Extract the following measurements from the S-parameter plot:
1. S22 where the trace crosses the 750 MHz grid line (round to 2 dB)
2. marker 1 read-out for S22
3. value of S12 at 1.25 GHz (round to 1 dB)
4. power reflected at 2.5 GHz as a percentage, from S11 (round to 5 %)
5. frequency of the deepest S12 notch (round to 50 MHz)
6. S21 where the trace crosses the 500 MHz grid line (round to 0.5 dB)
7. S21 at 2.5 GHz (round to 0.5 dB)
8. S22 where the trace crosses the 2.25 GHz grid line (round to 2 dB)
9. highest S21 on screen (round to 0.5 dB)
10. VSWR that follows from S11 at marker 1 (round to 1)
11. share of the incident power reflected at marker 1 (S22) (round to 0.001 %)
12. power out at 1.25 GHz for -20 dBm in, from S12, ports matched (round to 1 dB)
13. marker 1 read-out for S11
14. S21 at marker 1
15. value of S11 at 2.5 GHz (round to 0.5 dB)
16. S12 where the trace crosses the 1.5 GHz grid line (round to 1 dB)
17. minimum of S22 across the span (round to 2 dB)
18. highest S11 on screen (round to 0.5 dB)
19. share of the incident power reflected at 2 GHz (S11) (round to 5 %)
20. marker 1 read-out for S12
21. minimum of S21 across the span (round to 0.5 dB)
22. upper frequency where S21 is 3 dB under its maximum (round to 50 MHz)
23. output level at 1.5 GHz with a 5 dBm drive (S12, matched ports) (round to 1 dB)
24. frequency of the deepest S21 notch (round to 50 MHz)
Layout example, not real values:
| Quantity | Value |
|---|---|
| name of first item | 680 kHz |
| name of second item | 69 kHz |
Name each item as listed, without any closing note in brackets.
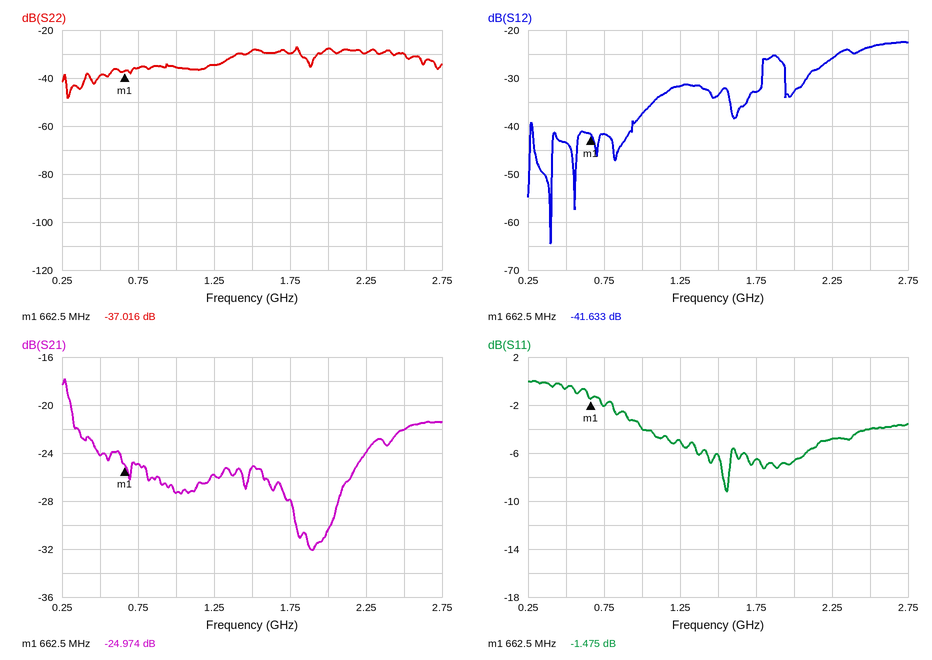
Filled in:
| Quantity | Value |
|---|---|
| S22 where the trace crosses the 750 MHz grid line | -36 dB |
| marker 1 read-out for S22 | -37.016 dB |
| value of S12 at 1.25 GHz | -32 dB |
| power reflected at 2.5 GHz as a percentage, from S11 | 40 % |
| frequency of the deepest S12 notch | 400 MHz |
| S21 where the trace crosses the 500 MHz grid line | -24.0 dB |
| S21 at 2.5 GHz | -22.0 dB |
| S22 where the trace crosses the 2.25 GHz grid line | -30 dB |
| highest S21 on screen | -18.0 dB |
| VSWR that follows from S11 at marker 1 | 12 |
| share of the incident power reflected at marker 1 (S22) | 0.020 % |
| power out at 1.25 GHz for -20 dBm in, from S12, ports matched | -52 dBm |
| marker 1 read-out for S11 | -1.475 dB |
| S21 at marker 1 | -24.974 dB |
| value of S11 at 2.5 GHz | -4.0 dB |
| S12 where the trace crosses the 1.5 GHz grid line | -34 dB |
| minimum of S22 across the span | -48 dB |
| highest S11 on screen | 0.0 dB |
| share of the incident power reflected at 2 GHz (S11) | 20 % |
| marker 1 read-out for S12 | -41.633 dB |
| minimum of S21 across the span | -32.0 dB |
| upper frequency where S21 is 3 dB under its maximum | 300 MHz |
| output level at 1.5 GHz with a 5 dBm drive (S12, matched ports) | -29 dBm |
| frequency of the deepest S21 notch | 1.90 GHz |
